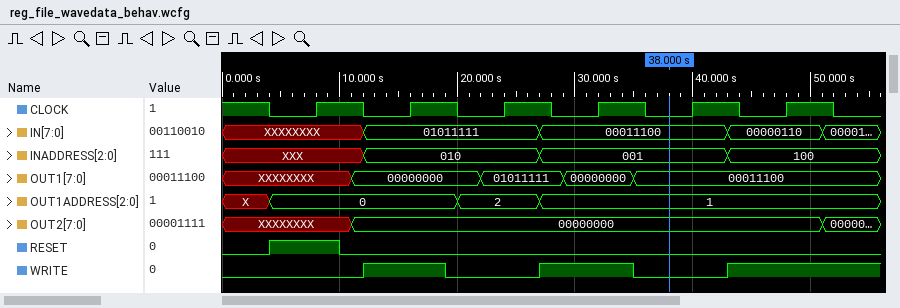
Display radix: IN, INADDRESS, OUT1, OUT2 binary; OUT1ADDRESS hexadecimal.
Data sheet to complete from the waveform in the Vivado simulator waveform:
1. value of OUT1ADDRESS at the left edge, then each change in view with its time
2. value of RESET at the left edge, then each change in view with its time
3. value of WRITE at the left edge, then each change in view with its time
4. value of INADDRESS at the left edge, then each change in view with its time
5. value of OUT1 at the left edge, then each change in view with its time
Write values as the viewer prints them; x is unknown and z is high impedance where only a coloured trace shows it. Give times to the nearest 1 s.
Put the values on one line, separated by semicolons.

X, 0 at 4 s, 2 at 20 s, 1 at 27 s; 0, 1 at 4 s, 0 at 10 s; 0, 1 at 12 s, 0 at 19 s, 1 at 27 s, 0 at 35 s, 1 at 43 s; XXX, 010 at 12 s, 001 at 27 s, 100 at 43 s; XXXXXXXX, 00000000 at 11 s, 01011111 at 22 s, 00000000 at 29 s, 00011100 at 35 s
